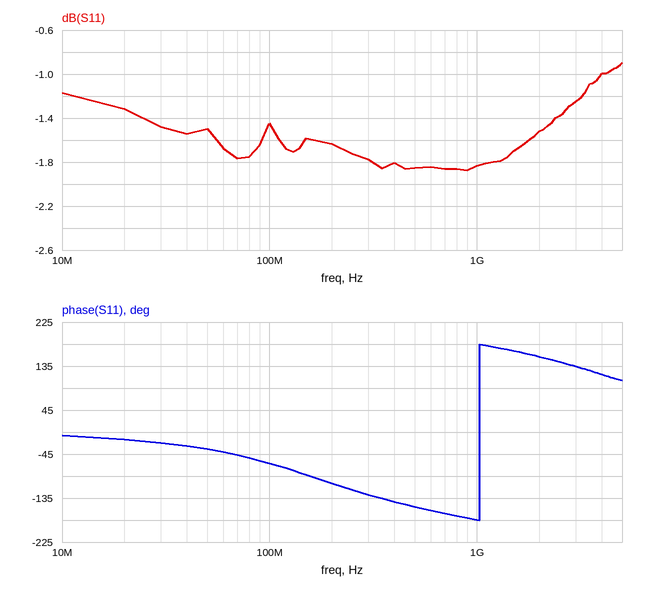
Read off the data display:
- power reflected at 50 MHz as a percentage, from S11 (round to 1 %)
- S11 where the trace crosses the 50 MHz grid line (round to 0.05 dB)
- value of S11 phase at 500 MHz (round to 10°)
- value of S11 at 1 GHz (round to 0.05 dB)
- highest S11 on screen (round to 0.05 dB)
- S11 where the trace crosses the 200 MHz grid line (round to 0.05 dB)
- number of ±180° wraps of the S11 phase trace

71 %
-1.50 dB
-150°
-1.85 dB
-0.90 dB
-1.65 dB
1
